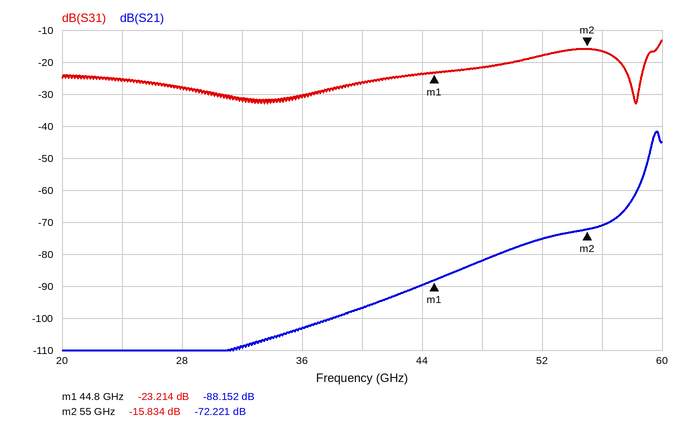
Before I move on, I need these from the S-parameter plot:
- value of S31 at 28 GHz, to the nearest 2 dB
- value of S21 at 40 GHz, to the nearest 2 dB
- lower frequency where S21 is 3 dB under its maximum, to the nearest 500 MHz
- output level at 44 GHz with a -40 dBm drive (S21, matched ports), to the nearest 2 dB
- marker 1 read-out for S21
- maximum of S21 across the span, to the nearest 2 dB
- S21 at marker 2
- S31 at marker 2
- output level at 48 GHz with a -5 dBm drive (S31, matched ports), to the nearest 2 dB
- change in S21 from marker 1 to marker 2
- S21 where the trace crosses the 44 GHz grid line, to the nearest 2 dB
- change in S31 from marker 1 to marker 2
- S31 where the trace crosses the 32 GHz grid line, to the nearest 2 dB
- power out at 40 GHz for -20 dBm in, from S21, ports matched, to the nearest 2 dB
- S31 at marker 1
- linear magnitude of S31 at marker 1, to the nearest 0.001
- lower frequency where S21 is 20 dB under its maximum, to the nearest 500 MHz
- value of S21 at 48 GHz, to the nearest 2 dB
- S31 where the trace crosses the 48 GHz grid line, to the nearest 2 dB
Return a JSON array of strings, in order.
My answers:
["-28 dB", "-96 dB", "59.5 GHz", "-130 dBm", "-88.152 dB", "-42 dB", "-72.221 dB", "-15.834 dB", "-26 dBm", "15.931 dB", "-90 dB", "7.380 dB", "-32 dB", "-116 dBm", "-23.214 dB", "0.069", "58.0 GHz", "-82 dB", "-22 dB"]
